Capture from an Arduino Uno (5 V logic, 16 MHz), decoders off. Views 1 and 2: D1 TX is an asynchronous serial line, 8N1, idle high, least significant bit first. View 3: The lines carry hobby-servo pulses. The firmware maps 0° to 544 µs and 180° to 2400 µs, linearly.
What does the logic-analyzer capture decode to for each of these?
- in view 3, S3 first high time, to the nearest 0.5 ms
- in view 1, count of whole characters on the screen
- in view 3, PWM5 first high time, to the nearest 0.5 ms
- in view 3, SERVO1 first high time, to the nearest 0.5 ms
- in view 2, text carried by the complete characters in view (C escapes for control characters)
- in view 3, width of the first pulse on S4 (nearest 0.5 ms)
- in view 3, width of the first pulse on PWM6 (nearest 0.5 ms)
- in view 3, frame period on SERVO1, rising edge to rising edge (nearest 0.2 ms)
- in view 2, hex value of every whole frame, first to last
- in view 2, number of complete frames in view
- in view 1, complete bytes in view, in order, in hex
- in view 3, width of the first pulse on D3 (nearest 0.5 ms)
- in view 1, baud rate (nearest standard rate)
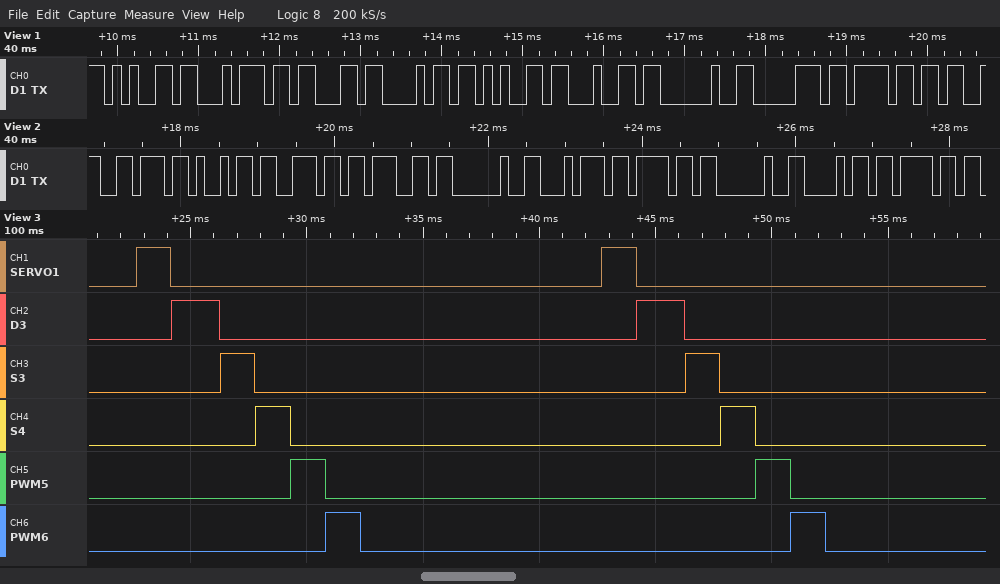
1.5 ms
9
1.5 ms
1.5 ms
"ving to ho"
1.5 ms
1.5 ms
20.0 ms
76 69 6E 67 20 74 6F 20 68 6F
10
65 74 63 68 65 64 20 70 6F
2.0 ms
9600 baud
